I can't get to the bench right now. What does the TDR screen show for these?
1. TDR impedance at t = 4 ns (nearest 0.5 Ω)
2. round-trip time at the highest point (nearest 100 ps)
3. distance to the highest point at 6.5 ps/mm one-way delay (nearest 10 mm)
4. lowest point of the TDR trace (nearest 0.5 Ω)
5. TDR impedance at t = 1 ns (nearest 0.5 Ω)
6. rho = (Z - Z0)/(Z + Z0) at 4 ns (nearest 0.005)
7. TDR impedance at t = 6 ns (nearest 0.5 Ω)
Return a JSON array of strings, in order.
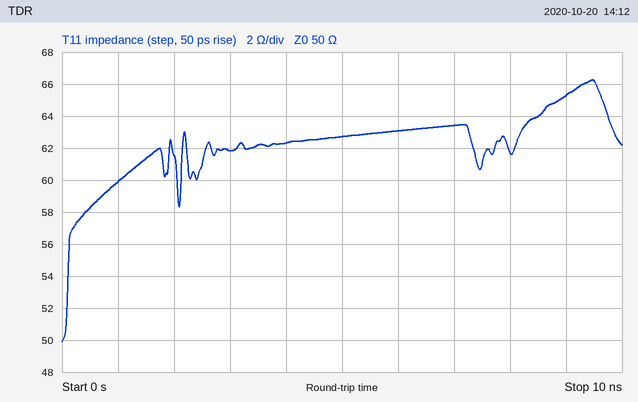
["62.5 Ω", "9.5 ns", "730 mm", "50.0 Ω", "60.0 Ω", "+0.110", "63.0 Ω"]
